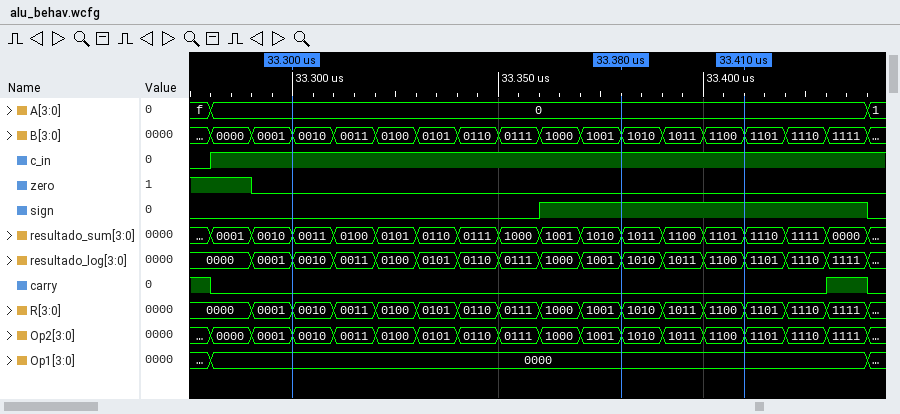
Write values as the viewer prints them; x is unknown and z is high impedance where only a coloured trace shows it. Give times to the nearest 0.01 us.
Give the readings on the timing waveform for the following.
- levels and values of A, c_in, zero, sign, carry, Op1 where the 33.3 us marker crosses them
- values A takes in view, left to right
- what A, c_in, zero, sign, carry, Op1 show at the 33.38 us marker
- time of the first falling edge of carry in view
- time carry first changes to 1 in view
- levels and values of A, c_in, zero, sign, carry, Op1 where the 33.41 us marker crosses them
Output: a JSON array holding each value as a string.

["A=0, c_in=1, zero=0, sign=0, carry=0, Op1=0000", "f, 0, 1", "A=0, c_in=1, zero=0, sign=1, carry=0, Op1=0000", "33.28 us", "33.43 us", "A=0, c_in=1, zero=0, sign=1, carry=0, Op1=0000"]
